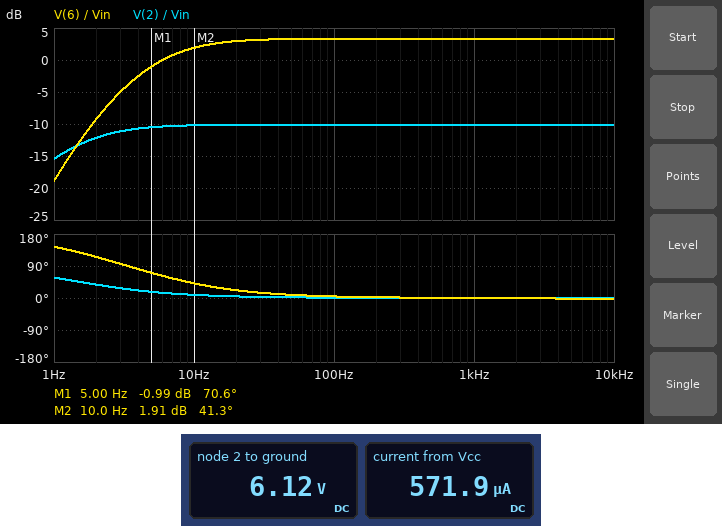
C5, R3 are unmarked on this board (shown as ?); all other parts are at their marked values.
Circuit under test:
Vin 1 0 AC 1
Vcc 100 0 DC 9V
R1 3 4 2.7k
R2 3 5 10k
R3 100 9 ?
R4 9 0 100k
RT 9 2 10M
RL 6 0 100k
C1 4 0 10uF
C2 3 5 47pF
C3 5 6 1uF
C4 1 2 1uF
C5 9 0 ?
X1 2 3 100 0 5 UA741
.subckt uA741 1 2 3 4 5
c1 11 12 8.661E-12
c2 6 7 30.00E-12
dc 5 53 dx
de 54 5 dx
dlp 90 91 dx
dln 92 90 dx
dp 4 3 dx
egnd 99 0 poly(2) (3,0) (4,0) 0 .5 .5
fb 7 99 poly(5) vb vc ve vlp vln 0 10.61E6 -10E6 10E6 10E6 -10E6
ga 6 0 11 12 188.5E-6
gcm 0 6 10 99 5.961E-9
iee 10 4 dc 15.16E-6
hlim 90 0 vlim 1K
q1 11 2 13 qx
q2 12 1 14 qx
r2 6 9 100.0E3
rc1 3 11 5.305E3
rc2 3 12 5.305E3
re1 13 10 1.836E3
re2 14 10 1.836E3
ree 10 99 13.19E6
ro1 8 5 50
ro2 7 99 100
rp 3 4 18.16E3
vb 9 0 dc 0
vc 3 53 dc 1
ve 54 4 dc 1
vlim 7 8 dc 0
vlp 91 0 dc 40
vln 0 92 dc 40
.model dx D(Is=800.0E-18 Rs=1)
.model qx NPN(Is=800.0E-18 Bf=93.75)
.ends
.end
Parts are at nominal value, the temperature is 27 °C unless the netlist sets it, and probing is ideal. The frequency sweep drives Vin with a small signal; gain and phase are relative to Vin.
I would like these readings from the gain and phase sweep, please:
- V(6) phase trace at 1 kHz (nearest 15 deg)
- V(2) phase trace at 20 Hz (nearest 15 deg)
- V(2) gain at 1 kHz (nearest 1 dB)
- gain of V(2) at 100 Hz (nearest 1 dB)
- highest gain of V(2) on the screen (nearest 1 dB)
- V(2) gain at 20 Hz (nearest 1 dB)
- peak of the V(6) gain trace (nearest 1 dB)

0 deg
0 deg
-10 dB
-10 dB
-10 dB
-10 dB
3 dB
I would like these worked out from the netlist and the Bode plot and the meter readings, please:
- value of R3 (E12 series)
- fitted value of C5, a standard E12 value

47 kΩ
2.2 µF
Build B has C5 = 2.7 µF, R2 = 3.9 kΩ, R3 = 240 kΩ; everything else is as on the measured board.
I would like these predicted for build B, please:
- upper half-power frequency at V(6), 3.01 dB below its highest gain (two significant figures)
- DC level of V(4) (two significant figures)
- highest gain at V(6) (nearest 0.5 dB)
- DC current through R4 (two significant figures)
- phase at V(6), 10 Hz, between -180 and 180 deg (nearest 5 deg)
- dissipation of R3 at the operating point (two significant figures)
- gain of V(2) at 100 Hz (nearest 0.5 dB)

360 kHz
2.6 V
-3.5 dB
26 µA
30 deg
170 µW
-11.5 dB
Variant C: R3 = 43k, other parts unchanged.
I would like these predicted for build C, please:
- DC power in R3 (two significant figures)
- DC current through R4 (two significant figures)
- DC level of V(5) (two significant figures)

170 µW
63 µA
6.3 V
